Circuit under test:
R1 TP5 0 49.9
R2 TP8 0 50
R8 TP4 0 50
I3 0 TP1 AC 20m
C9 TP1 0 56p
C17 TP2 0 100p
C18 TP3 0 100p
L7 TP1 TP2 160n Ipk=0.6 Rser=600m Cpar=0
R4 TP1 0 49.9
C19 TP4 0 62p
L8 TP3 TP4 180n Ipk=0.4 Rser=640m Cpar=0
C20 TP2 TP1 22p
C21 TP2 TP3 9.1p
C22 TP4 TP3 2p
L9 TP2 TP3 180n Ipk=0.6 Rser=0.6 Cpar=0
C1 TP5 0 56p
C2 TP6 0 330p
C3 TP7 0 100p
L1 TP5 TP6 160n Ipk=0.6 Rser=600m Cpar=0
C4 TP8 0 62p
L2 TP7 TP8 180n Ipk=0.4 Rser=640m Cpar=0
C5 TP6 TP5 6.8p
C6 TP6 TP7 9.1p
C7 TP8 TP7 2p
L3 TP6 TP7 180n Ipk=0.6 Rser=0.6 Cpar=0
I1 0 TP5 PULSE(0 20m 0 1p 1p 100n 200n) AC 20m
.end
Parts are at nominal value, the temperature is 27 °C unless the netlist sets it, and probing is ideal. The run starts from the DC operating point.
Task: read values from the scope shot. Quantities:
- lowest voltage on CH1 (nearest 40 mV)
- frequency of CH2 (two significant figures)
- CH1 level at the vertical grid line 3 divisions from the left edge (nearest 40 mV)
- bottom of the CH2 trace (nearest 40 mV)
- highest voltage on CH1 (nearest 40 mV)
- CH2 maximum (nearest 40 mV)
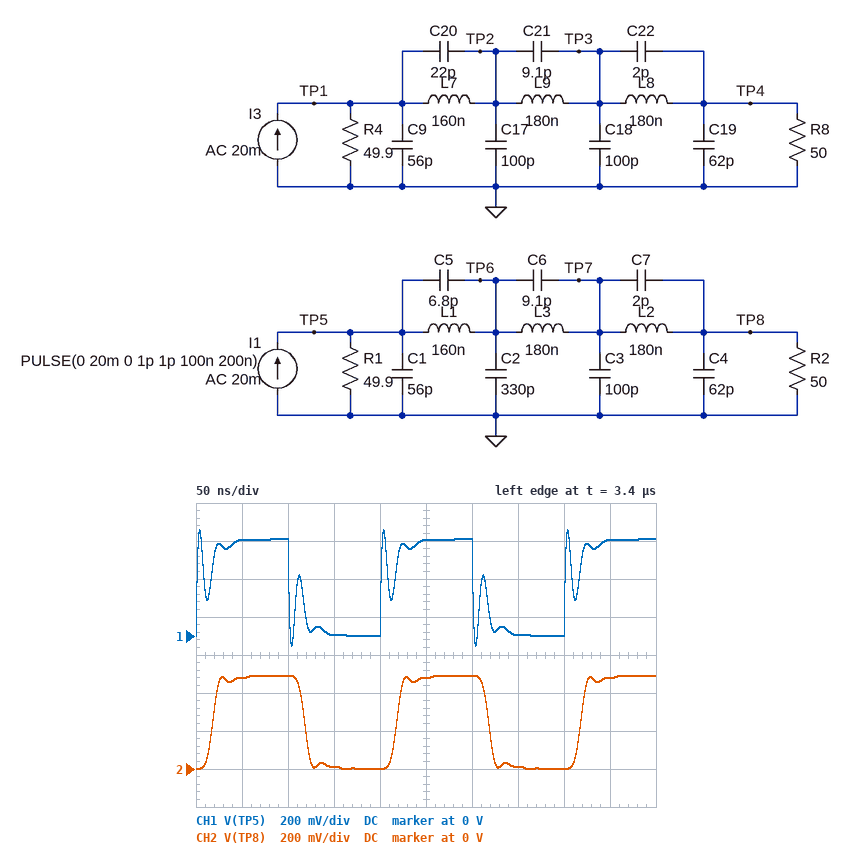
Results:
-40 mV
5.0 MHz
0 V
0 V
560 mV
480 mV
